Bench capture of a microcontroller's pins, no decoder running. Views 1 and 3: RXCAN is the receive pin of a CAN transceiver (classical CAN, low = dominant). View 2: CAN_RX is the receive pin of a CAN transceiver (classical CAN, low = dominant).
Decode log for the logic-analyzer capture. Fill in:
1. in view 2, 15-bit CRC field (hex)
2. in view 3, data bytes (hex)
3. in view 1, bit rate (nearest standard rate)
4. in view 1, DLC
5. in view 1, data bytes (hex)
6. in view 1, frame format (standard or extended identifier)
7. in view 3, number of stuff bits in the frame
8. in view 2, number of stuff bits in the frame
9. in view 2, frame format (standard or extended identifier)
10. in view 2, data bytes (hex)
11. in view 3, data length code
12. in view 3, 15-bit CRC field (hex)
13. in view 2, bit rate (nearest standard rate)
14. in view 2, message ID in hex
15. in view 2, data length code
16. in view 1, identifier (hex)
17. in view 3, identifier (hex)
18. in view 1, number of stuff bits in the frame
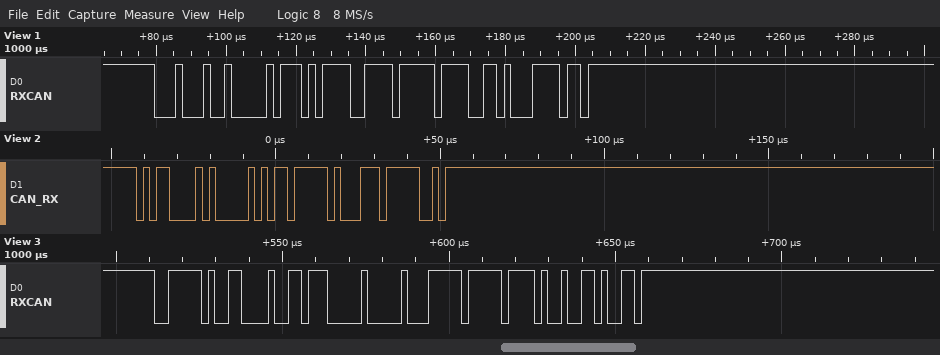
0x63BE
DC 00 1F FF
500 kbit/s
3
AF 3D FF
standard
5
3
standard
6F
4
0x5269
500 kbit/s
0x585
1
0x112
0x3F3
2
